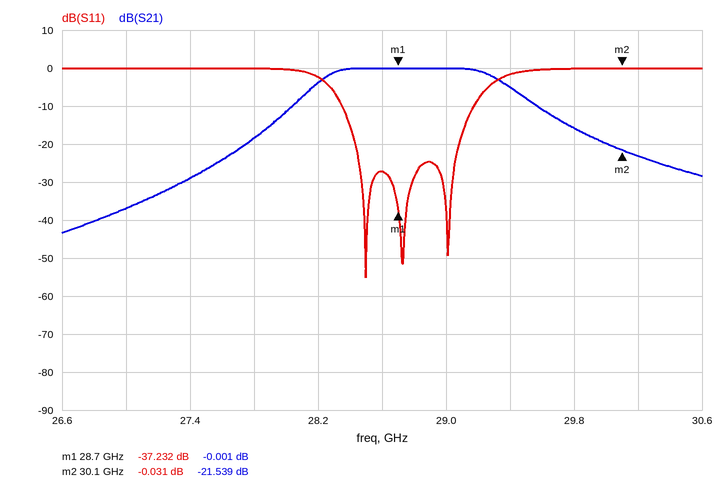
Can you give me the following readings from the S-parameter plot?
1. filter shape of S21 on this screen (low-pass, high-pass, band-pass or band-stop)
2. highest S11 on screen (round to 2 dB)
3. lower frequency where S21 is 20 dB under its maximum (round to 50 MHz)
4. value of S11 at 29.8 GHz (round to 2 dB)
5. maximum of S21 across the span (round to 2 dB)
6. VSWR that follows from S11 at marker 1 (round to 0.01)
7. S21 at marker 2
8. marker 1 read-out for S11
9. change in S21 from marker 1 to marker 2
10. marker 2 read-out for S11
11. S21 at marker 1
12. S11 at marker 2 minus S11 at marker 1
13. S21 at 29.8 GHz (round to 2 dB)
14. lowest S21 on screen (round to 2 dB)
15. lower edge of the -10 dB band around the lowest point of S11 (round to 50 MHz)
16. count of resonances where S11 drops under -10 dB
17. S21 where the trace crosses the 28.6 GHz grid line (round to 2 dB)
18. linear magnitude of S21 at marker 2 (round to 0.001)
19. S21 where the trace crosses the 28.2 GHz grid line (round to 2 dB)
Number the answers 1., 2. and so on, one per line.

1. band-pass
2. 0 dB
3. 27.75 GHz
4. 0 dB
5. 0 dB
6. 1.03
7. -21.539 dB
8. -37.232 dB
9. -21.538 dB
10. -0.031 dB
11. -0.001 dB
12. 37.201 dB
13. -16 dB
14. -44 dB
15. 28.35 GHz
16. 3
17. 0 dB
18. 0.084
19. -4 dB
